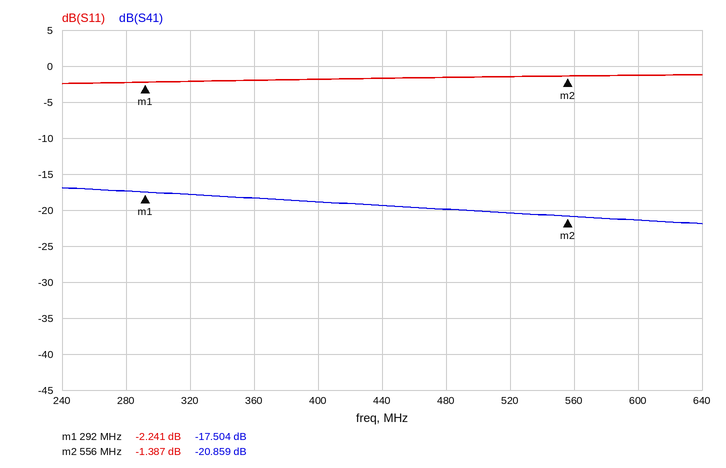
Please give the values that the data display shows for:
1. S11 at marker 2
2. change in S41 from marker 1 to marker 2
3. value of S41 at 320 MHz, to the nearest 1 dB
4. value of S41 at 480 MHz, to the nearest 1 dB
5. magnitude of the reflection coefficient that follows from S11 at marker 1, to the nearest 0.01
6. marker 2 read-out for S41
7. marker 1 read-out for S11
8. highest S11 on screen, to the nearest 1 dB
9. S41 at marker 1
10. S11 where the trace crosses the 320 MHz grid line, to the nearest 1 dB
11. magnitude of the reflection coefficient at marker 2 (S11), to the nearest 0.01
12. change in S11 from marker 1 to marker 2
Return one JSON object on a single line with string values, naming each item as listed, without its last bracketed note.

{"S11 at marker 2": "-1.387 dB", "change in S41 from marker 1 to marker 2": "-3.355 dB", "value of S41 at 320 MHz, to the nearest 1 dB": "-18 dB", "value of S41 at 480 MHz, to the nearest 1 dB": "-20 dB", "magnitude of the reflection coefficient that follows from S11 at marker 1, to the nearest 0.01": "0.77", "marker 2 read-out for S41": "-20.859 dB", "marker 1 read-out for S11": "-2.241 dB", "highest S11 on screen, to the nearest 1 dB": "-1 dB", "S41 at marker 1": "-17.504 dB", "S11 where the trace crosses the 320 MHz grid line, to the nearest 1 dB": "-2 dB", "magnitude of the reflection coefficient at marker 2 (S11), to the nearest 0.01": "0.85", "change in S11 from marker 1 to marker 2": "0.854 dB"}
